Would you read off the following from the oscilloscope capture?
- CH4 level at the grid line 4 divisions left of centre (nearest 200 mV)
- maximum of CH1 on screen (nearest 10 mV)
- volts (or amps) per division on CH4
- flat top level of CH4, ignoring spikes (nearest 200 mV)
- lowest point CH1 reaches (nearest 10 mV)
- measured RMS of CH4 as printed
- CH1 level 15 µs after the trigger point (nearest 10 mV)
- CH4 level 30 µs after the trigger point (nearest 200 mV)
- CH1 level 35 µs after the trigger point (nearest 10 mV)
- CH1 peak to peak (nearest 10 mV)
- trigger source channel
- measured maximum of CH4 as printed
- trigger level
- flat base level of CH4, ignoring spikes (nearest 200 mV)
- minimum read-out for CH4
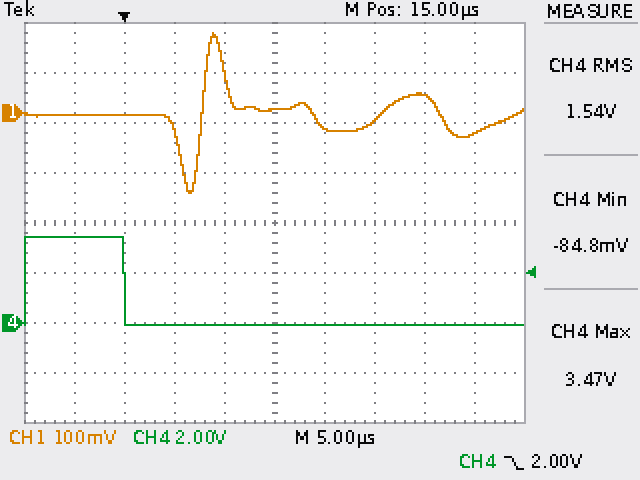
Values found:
3.4 V
160 mV
2 V
3.4 V
-160 mV
1.54 V
10 mV
0.0 V
-40 mV
320 mV
CH4
3.47 V
2.00 V
0.0 V
-84.8 mV
